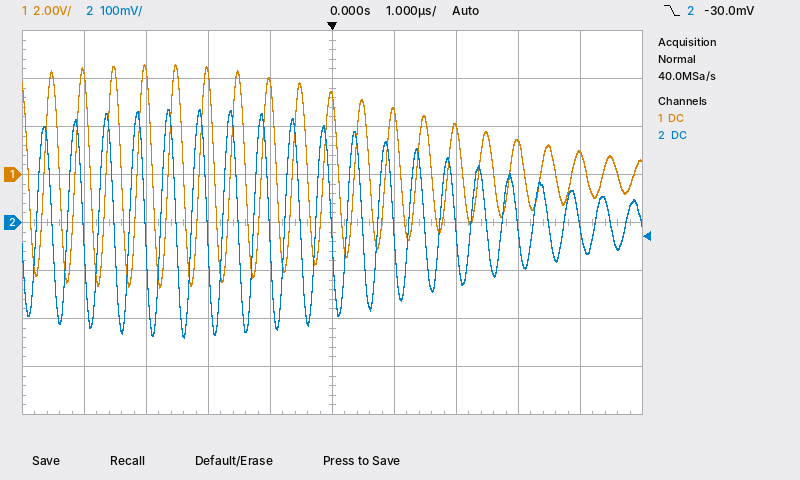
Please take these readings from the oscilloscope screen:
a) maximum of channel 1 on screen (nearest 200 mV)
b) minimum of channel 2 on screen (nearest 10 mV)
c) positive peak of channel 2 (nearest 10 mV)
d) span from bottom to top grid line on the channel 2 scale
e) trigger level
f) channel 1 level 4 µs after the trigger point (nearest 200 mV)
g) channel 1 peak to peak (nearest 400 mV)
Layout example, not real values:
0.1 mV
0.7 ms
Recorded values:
4.6 V
-240 mV
240 mV
800 mV
-30.0 mV
800 mV
9.2 V
